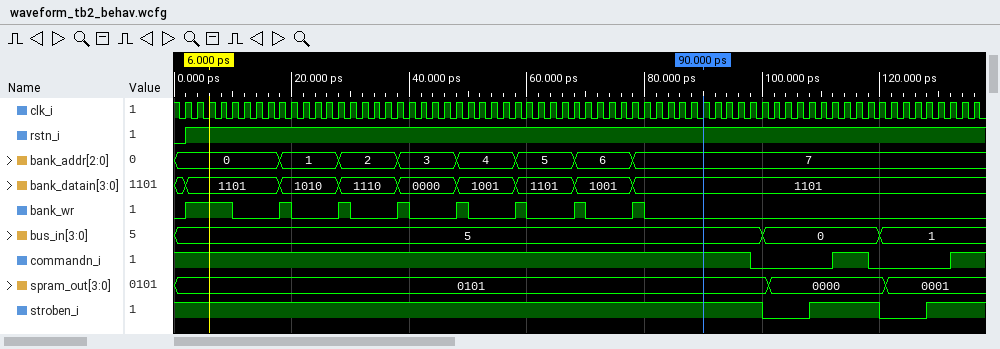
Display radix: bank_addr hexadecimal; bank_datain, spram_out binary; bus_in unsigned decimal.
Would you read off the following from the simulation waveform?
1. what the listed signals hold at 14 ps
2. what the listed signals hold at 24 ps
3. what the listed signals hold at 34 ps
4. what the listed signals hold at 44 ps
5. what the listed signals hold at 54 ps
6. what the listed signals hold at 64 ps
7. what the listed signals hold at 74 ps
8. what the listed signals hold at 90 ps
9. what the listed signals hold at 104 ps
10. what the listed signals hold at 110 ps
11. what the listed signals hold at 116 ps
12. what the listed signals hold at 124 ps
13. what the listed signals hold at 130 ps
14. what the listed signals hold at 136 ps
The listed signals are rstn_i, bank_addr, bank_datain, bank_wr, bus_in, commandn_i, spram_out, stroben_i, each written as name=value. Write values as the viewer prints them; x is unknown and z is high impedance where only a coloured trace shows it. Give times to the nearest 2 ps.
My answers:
rstn_i=1, bank_addr=0, bank_datain=1101, bank_wr=0, bus_in=5, commandn_i=1, spram_out=0101, stroben_i=1
rstn_i=1, bank_addr=1, bank_datain=1010, bank_wr=0, bus_in=5, commandn_i=1, spram_out=0101, stroben_i=1
rstn_i=1, bank_addr=2, bank_datain=1110, bank_wr=0, bus_in=5, commandn_i=1, spram_out=0101, stroben_i=1
rstn_i=1, bank_addr=3, bank_datain=0000, bank_wr=0, bus_in=5, commandn_i=1, spram_out=0101, stroben_i=1
rstn_i=1, bank_addr=4, bank_datain=1001, bank_wr=0, bus_in=5, commandn_i=1, spram_out=0101, stroben_i=1
rstn_i=1, bank_addr=5, bank_datain=1101, bank_wr=0, bus_in=5, commandn_i=1, spram_out=0101, stroben_i=1
rstn_i=1, bank_addr=6, bank_datain=1001, bank_wr=0, bus_in=5, commandn_i=1, spram_out=0101, stroben_i=1
rstn_i=1, bank_addr=7, bank_datain=1101, bank_wr=0, bus_in=5, commandn_i=1, spram_out=0101, stroben_i=1
rstn_i=1, bank_addr=7, bank_datain=1101, bank_wr=0, bus_in=0, commandn_i=0, spram_out=0000, stroben_i=0
rstn_i=1, bank_addr=7, bank_datain=1101, bank_wr=0, bus_in=0, commandn_i=0, spram_out=0000, stroben_i=1
rstn_i=1, bank_addr=7, bank_datain=1101, bank_wr=0, bus_in=0, commandn_i=1, spram_out=0000, stroben_i=1
rstn_i=1, bank_addr=7, bank_datain=1101, bank_wr=0, bus_in=1, commandn_i=0, spram_out=0001, stroben_i=0
rstn_i=1, bank_addr=7, bank_datain=1101, bank_wr=0, bus_in=1, commandn_i=0, spram_out=0001, stroben_i=1
rstn_i=1, bank_addr=7, bank_datain=1101, bank_wr=0, bus_in=1, commandn_i=1, spram_out=0001, stroben_i=1
